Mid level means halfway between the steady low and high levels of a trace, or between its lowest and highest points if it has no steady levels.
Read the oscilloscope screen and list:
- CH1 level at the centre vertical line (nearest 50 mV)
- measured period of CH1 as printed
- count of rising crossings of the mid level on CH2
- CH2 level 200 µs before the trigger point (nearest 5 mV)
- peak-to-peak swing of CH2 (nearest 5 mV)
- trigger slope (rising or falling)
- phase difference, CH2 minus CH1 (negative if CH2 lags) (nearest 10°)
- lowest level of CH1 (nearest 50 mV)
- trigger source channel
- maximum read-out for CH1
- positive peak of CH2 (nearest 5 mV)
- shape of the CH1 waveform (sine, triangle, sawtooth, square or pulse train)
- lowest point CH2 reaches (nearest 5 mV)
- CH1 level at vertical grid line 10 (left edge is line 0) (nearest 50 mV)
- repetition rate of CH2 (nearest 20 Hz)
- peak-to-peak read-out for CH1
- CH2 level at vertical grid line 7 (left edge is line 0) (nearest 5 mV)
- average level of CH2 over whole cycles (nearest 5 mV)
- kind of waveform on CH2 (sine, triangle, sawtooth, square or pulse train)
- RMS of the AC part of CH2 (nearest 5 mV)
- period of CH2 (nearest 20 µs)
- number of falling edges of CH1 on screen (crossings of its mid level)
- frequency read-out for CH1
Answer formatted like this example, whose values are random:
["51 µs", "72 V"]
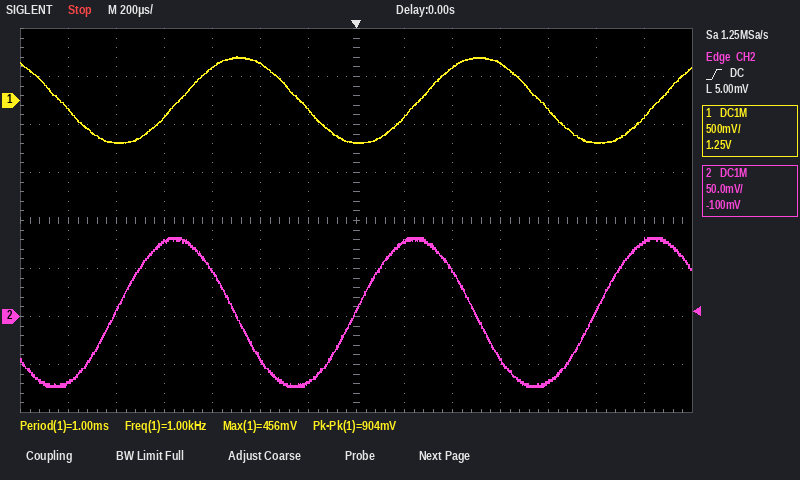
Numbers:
["-450 mV", "1.00 ms", "3", "-70 mV", "155 mV", "rising", "+100°", "-450 mV", "CH2", "456 mV", "80 mV", "sine", "-75 mV", "400 mV", "1.00 kHz", "904 mV", "5 mV", "5 mV", "sine", "55 mV", "1.00 ms", "3", "1.00 kHz"]
